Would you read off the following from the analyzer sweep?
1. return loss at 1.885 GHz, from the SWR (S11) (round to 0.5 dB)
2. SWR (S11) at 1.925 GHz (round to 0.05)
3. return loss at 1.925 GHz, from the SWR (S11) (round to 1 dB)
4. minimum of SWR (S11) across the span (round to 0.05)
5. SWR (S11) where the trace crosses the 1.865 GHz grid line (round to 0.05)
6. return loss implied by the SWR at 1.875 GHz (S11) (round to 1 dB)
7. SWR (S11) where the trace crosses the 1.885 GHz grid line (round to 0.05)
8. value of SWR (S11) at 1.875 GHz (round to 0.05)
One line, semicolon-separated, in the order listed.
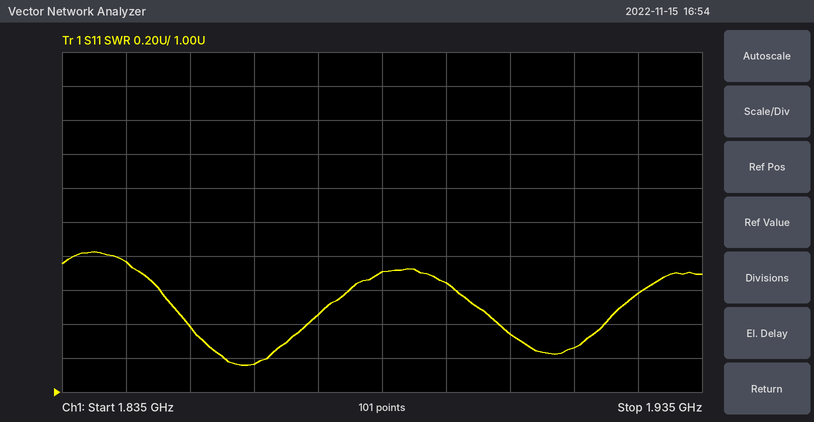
11.5 dB; 1.60; 13 dB; 1.15; 1.15; 15 dB; 1.70; 1.45
